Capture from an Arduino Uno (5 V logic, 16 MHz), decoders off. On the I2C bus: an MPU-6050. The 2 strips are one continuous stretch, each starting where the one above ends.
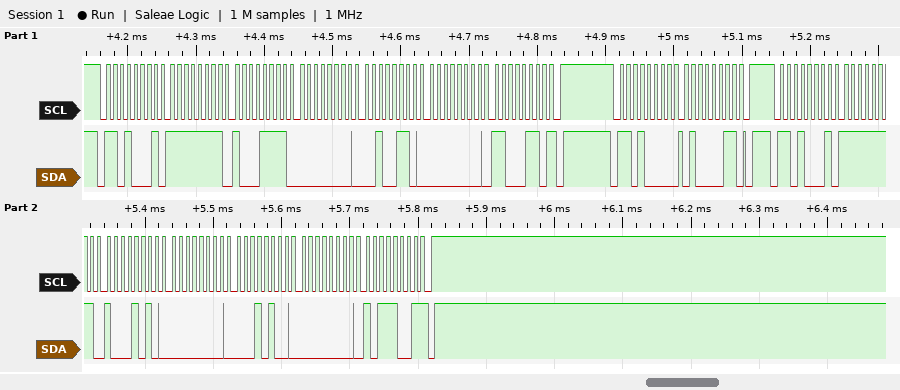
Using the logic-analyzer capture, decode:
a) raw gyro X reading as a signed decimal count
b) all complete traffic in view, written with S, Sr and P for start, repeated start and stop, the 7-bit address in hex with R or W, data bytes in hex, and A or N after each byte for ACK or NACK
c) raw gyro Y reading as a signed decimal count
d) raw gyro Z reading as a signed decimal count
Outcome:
-118
S 68R A FF A 8F A 00 A 26 A 00 A C6 N P S 68W A 43 A P S 68R A FF A 8A A 00 A 14 A 00 A B9 N P
20
185
